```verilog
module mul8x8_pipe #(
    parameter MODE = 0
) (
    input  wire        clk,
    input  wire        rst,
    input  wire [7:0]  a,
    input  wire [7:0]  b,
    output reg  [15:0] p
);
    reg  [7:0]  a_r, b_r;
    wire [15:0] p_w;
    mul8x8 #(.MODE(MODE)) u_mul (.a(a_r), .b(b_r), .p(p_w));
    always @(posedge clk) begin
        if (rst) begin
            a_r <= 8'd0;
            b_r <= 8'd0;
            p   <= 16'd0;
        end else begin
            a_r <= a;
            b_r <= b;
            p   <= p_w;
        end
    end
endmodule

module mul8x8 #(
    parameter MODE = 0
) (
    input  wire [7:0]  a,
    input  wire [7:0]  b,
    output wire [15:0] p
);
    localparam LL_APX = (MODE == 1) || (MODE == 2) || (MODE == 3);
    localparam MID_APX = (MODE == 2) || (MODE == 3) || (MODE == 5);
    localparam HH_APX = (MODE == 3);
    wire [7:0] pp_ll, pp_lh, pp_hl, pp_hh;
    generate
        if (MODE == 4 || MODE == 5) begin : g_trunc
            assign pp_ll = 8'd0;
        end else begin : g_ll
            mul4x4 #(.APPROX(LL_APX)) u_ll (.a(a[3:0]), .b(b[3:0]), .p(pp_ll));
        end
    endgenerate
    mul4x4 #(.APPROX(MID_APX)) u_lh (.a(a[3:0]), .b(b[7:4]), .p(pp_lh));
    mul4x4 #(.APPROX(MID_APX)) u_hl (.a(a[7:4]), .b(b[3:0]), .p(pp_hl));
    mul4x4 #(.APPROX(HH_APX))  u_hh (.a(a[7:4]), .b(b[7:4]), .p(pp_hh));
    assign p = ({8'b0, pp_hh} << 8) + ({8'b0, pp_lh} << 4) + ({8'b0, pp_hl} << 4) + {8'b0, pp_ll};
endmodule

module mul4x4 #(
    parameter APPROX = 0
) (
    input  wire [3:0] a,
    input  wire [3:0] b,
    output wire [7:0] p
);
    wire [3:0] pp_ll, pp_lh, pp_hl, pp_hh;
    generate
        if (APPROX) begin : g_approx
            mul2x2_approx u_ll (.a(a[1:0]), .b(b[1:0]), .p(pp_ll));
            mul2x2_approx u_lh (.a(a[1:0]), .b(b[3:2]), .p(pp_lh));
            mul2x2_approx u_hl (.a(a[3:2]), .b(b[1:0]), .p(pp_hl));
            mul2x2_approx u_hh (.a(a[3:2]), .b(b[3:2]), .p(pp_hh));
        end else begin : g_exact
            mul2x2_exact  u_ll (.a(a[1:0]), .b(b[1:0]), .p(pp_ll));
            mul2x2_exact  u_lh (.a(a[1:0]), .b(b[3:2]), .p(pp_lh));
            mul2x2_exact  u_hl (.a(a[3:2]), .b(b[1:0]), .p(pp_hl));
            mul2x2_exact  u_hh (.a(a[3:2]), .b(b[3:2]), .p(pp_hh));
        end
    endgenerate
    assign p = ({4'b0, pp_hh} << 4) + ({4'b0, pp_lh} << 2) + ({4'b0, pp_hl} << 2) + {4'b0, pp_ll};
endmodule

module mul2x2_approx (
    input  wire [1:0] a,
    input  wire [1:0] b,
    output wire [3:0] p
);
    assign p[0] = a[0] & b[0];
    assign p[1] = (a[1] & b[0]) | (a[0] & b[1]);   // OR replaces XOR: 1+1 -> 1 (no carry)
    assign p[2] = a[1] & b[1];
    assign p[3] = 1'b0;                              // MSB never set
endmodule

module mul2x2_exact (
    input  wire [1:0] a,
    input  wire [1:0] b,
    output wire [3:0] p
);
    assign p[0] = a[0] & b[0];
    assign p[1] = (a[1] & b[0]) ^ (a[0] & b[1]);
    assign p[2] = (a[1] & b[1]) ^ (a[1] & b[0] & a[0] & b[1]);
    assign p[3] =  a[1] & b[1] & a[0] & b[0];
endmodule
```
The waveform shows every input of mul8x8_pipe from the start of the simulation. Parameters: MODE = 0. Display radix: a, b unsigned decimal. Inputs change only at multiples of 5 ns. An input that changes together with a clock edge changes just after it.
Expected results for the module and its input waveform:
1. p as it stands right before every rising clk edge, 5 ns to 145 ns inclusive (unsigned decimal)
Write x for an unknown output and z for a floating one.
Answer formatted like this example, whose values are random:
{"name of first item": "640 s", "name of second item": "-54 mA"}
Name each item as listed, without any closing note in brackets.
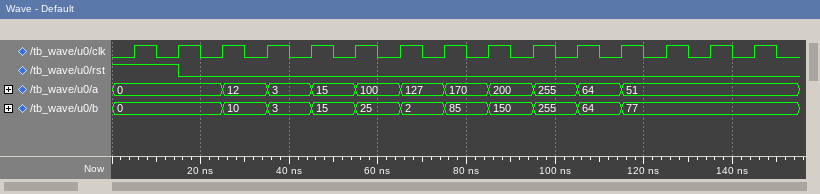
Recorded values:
{"p as it stands right before every rising clk edge, 5 ns to 145 ns inclusive": "x, 0, 0, 0, 0, 120, 9, 225, 2500, 254, 14450, 30000, 65025, 4096, 3927"}
